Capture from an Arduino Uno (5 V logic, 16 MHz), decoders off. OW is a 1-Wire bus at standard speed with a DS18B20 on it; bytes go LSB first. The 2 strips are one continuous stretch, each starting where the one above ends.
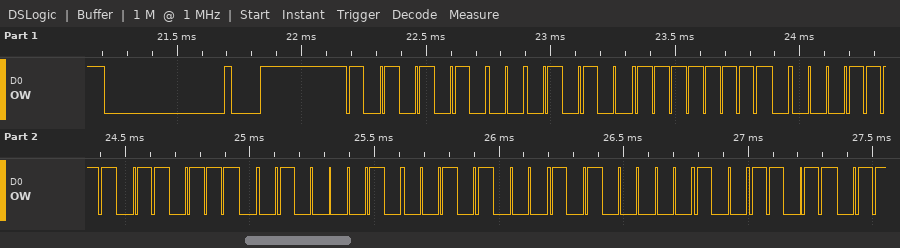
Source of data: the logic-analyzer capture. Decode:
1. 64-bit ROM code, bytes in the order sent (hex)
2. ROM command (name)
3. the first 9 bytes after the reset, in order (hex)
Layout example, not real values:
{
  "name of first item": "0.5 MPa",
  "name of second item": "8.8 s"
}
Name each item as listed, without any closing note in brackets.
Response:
{
  "64-bit ROM code, bytes in the order sent": "28 FF F0 76 42 14 05 D9",
  "ROM command": "Match ROM",
  "the first 9 bytes after the reset, in order": "55 28 FF F0 76 42 14 05 D9"
}
